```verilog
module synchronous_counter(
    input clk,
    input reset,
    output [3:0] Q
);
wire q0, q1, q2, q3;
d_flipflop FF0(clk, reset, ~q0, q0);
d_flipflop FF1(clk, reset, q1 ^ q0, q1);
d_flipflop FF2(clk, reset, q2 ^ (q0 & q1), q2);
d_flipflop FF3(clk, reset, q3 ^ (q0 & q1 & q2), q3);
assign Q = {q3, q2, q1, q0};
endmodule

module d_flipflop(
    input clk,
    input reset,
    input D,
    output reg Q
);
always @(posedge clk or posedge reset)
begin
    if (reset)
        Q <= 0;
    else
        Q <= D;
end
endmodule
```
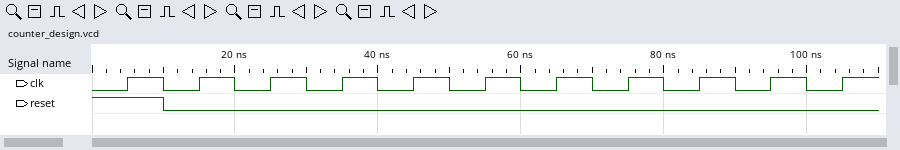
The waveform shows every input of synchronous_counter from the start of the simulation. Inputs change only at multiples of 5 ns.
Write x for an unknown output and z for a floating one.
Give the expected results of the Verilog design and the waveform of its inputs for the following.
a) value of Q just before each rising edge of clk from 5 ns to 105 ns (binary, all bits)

0000, 0000, 0001, 0010, 0011, 0100, 0101, 0110, 0111, 1000, 1001
